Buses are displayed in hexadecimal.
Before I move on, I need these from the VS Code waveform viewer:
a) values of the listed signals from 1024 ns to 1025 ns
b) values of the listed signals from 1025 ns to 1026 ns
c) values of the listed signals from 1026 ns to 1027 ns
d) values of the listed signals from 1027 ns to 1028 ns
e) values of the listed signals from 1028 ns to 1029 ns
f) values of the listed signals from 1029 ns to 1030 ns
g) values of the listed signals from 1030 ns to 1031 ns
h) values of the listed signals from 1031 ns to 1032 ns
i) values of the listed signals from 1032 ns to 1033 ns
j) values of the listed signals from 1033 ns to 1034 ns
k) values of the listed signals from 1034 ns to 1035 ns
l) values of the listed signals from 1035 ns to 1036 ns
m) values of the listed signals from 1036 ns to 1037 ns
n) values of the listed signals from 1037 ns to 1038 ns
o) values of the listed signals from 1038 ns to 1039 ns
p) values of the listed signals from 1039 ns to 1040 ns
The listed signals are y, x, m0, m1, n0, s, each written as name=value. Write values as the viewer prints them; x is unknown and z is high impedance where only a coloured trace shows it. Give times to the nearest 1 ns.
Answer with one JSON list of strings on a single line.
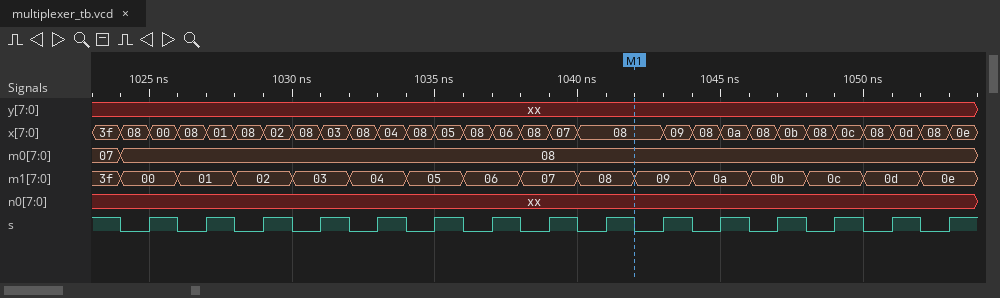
["y=xx, x=08, m0=08, m1=00, n0=xx, s=0", "y=xx, x=00, m0=08, m1=00, n0=xx, s=1", "y=xx, x=08, m0=08, m1=01, n0=xx, s=0", "y=xx, x=01, m0=08, m1=01, n0=xx, s=1", "y=xx, x=08, m0=08, m1=02, n0=xx, s=0", "y=xx, x=02, m0=08, m1=02, n0=xx, s=1", "y=xx, x=08, m0=08, m1=03, n0=xx, s=0", "y=xx, x=03, m0=08, m1=03, n0=xx, s=1", "y=xx, x=08, m0=08, m1=04, n0=xx, s=0", "y=xx, x=04, m0=08, m1=04, n0=xx, s=1", "y=xx, x=08, m0=08, m1=05, n0=xx, s=0", "y=xx, x=05, m0=08, m1=05, n0=xx, s=1", "y=xx, x=08, m0=08, m1=06, n0=xx, s=0", "y=xx, x=06, m0=08, m1=06, n0=xx, s=1", "y=xx, x=08, m0=08, m1=07, n0=xx, s=0", "y=xx, x=07, m0=08, m1=07, n0=xx, s=1"]
